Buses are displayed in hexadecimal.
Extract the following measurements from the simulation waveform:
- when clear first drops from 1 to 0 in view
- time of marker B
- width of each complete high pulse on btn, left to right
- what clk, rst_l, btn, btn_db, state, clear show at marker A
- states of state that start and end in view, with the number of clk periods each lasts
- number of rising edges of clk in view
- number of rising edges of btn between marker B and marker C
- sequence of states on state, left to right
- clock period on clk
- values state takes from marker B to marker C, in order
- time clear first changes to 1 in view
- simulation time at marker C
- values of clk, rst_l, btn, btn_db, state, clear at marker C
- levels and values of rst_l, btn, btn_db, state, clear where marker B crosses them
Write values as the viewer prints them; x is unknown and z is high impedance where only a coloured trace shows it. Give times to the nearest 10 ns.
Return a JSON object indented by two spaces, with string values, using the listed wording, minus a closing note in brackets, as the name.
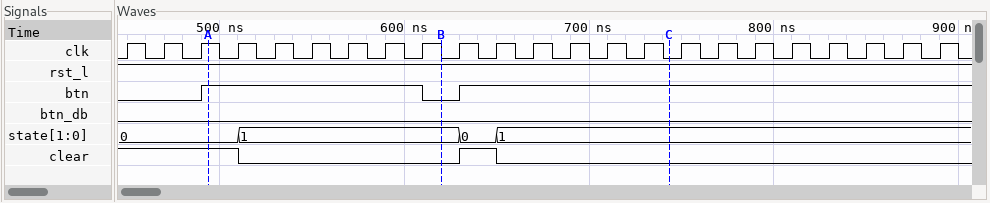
{
  "when clear first drops from 1 to 0 in view": "510 ns",
  "time of marker B": "620 ns",
  "width of each complete high pulse on btn, left to right": "120 ns",
  "what clk, rst_l, btn, btn_db, state, clear show at marker A": "clk=1, rst_l=1, btn=1, btn_db=0, state=0, clear=1",
  "states of state that start and end in view, with the number of clk periods each lasts": "1: 6, 0: 1",
  "number of rising edges of clk in view": "23",
  "number of rising edges of btn between marker B and marker C": "1",
  "sequence of states on state, left to right": "0, 1, 0, 1",
  "clock period on clk": "20 ns",
  "values state takes from marker B to marker C, in order": "1, 0, 1",
  "time clear first changes to 1 in view": "630 ns",
  "simulation time at marker C": "740 ns",
  "values of clk, rst_l, btn, btn_db, state, clear at marker C": "clk=0, rst_l=1, btn=1, btn_db=0, state=1, clear=0",
  "levels and values of rst_l, btn, btn_db, state, clear where marker B crosses them": "rst_l=1, btn=0, btn_db=0, state=1, clear=0"
}
